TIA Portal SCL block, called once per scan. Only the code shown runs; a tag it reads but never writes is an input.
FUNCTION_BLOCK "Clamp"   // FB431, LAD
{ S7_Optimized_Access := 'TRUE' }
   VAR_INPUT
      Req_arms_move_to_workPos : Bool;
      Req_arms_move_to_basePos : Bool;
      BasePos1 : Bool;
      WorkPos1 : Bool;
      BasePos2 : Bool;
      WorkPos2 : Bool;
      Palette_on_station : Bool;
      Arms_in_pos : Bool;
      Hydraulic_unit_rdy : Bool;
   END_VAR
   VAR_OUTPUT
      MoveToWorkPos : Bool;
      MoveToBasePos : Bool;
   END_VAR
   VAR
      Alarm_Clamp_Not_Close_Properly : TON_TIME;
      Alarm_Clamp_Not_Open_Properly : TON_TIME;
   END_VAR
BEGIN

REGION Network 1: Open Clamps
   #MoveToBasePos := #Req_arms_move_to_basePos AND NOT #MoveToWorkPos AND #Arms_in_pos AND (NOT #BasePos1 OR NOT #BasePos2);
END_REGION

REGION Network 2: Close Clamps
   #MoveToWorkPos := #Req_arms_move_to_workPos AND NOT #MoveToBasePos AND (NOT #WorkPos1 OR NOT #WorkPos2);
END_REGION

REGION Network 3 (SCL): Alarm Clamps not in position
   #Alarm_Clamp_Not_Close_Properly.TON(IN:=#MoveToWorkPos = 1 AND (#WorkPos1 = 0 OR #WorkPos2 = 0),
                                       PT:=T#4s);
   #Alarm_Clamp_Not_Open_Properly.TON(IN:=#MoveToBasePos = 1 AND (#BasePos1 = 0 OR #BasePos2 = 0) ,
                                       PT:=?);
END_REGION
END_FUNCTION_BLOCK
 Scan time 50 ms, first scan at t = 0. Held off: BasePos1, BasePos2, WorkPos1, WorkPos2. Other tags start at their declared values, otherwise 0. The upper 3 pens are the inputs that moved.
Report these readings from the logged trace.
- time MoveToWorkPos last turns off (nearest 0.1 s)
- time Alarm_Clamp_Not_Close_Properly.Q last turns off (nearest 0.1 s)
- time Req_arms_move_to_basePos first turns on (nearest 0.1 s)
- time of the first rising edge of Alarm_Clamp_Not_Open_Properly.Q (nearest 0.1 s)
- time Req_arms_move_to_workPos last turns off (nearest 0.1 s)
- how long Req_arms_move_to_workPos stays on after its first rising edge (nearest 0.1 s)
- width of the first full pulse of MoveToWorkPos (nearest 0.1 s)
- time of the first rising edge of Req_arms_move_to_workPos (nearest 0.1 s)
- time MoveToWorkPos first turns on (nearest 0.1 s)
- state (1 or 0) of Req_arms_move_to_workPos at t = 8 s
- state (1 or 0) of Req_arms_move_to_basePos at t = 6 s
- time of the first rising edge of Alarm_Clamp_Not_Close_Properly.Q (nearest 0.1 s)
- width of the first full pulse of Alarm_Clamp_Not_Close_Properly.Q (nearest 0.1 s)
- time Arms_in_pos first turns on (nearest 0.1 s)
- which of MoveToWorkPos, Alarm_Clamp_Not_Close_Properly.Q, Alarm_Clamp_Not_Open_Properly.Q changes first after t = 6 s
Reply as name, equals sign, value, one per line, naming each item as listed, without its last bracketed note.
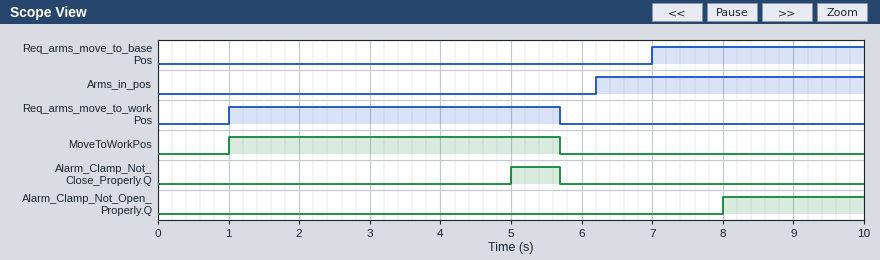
time MoveToWorkPos last turns off = 5.7 s
time Alarm_Clamp_Not_Close_Properly.Q last turns off = 5.7 s
time Req_arms_move_to_basePos first turns on = 7.0 s
time of the first rising edge of Alarm_Clamp_Not_Open_Properly.Q = 8.0 s
time Req_arms_move_to_workPos last turns off = 5.7 s
how long Req_arms_move_to_workPos stays on after its first rising edge = 4.7 s
width of the first full pulse of MoveToWorkPos = 4.7 s
time of the first rising edge of Req_arms_move_to_workPos = 1.0 s
time MoveToWorkPos first turns on = 1.0 s
state (1 or 0) of Req_arms_move_to_workPos at t = 8 s = 0
state (1 or 0) of Req_arms_move_to_basePos at t = 6 s = 0
time of the first rising edge of Alarm_Clamp_Not_Close_Properly.Q = 5.0 s
width of the first full pulse of Alarm_Clamp_Not_Close_Properly.Q = 0.7 s
time Arms_in_pos first turns on = 6.2 s
which of MoveToWorkPos, Alarm_Clamp_Not_Close_Properly.Q, Alarm_Clamp_Not_Open_Properly.Q changes first after t = 6 s = Alarm_Clamp_Not_Open_Properly.Q
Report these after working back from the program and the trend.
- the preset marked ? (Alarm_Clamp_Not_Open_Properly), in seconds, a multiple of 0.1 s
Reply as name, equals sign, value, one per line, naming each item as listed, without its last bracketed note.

the preset marked ? (Alarm_Clamp_Not_Open_Properly), in seconds, a multiple of 0.1 s = 1.0 s
